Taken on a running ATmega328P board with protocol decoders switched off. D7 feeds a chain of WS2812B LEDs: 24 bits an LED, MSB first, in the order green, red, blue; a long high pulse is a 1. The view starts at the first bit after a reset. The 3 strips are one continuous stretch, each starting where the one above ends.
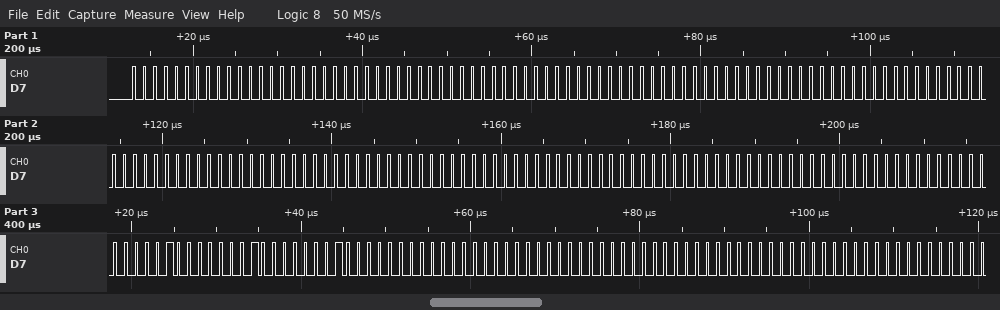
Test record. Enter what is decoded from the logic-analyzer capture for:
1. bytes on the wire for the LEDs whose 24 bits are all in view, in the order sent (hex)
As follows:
00 00 00 00 00 00 00 00 00 00 00 00 00 00 00 00 00 00 00 00 00 40 40 40 00 00 00 00 00 00
